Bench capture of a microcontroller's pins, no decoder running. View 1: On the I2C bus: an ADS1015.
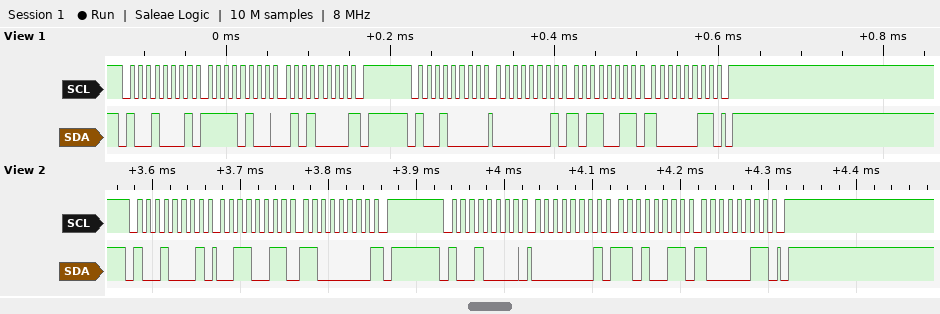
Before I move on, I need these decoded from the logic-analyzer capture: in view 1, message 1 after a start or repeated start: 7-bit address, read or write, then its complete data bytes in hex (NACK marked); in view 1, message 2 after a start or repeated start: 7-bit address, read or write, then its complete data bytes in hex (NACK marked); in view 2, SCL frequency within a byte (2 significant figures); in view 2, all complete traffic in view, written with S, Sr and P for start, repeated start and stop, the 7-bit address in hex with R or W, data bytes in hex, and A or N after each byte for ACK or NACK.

0x48 read: F4 50 NACK
0x48 write: 01 B3 83
100 kHz
S 48R A 33 A C0 N P S 48W A 01 A D3 A 83 A P
